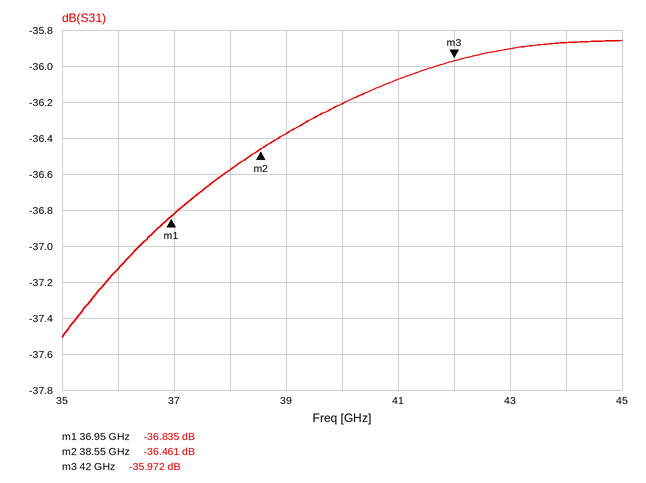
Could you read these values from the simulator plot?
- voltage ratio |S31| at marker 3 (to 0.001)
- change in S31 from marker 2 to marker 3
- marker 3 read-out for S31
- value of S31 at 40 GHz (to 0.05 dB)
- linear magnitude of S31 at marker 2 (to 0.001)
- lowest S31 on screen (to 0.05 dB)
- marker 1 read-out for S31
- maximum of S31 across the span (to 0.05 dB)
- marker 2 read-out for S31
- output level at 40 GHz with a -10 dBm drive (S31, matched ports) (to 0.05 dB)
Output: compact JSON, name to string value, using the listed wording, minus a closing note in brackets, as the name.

{"voltage ratio |S31| at marker 3": "0.016", "change in S31 from marker 2 to marker 3": "0.489 dB", "marker 3 read-out for S31": "-35.972 dB", "value of S31 at 40 GHz": "-36.20 dB", "linear magnitude of S31 at marker 2": "0.015", "lowest S31 on screen": "-37.50 dB", "marker 1 read-out for S31": "-36.835 dB", "maximum of S31 across the span": "-35.85 dB", "marker 2 read-out for S31": "-36.461 dB", "output level at 40 GHz with a -10 dBm drive (S31, matched ports)": "-46.20 dBm"}
